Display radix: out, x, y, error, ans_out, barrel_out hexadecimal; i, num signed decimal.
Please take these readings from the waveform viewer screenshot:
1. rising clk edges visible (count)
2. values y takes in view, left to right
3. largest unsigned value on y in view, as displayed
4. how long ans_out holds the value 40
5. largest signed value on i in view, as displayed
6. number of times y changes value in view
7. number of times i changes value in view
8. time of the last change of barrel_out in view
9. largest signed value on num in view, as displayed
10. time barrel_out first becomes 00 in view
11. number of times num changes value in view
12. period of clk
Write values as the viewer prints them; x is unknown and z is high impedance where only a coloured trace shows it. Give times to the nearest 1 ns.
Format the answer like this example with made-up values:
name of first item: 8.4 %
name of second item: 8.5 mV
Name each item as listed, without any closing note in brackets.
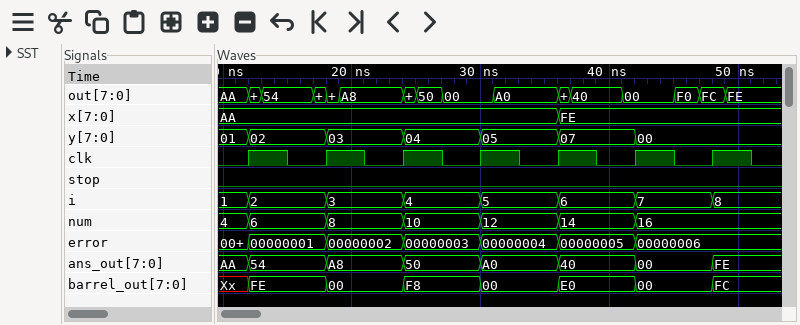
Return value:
rising clk edges visible: 7
values y takes in view, left to right: 01, 02, 03, 04, 05, 07, 00
largest unsigned value on y in view, as displayed: 07
how long ans_out holds the value 40: 6 ns
largest signed value on i in view, as displayed: 8
number of times y changes value in view: 6
number of times i changes value in view: 7
time of the last change of barrel_out in view: 48 ns
largest signed value on num in view, as displayed: 16
time barrel_out first becomes 00 in view: 18 ns
number of times num changes value in view: 6
period of clk: 6 ns
